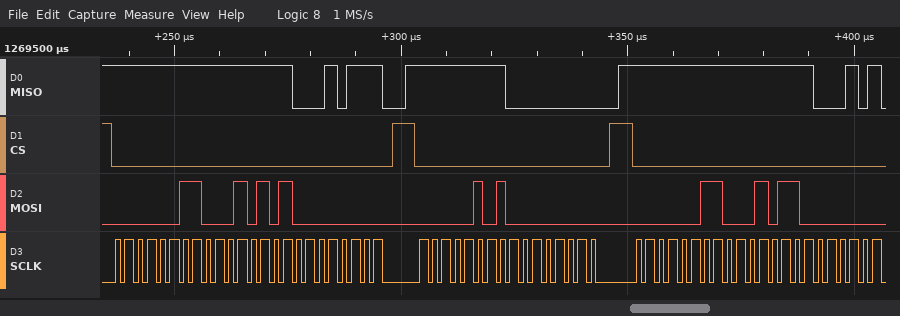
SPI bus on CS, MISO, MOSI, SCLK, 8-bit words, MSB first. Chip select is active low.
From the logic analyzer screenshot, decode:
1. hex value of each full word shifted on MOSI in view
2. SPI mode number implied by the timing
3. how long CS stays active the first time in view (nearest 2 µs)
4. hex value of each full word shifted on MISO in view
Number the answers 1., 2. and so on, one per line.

1. 03, 15, 00, 05, 00, 03, 16
2. 0
3. 62 µs
4. FF, FF, 17, FF, 00, FF, FF
